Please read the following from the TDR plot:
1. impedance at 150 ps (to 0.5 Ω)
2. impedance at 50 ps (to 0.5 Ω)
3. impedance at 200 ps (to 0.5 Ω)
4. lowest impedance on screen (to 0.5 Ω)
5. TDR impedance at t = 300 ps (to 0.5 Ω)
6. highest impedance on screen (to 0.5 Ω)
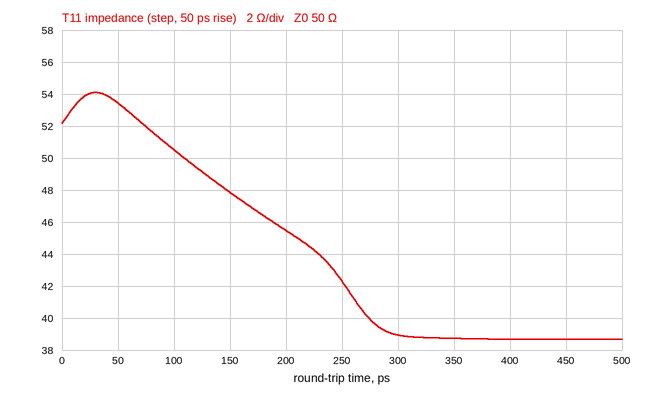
48.0 Ω
53.5 Ω
45.5 Ω
38.5 Ω
39.0 Ω
54.0 Ω
